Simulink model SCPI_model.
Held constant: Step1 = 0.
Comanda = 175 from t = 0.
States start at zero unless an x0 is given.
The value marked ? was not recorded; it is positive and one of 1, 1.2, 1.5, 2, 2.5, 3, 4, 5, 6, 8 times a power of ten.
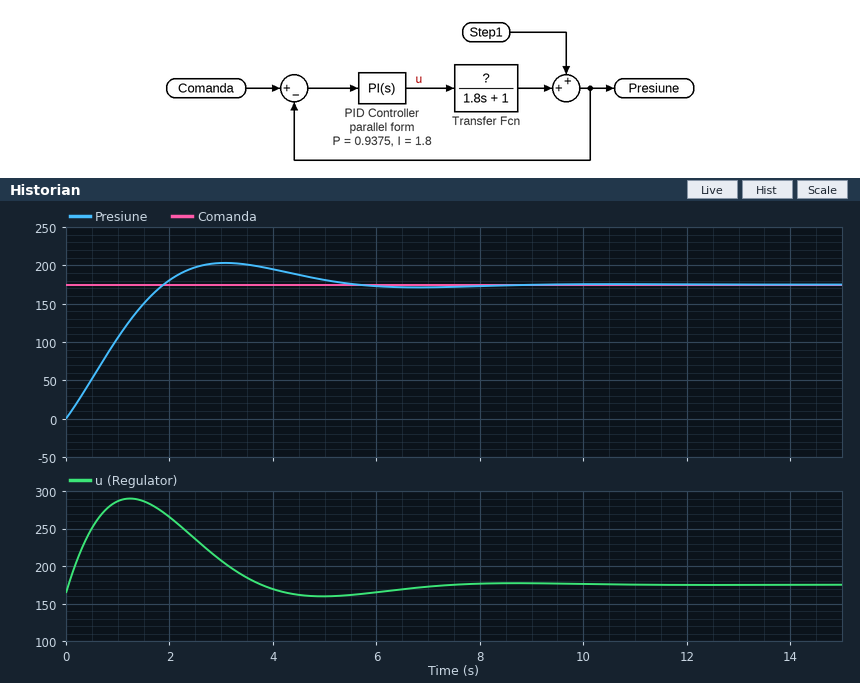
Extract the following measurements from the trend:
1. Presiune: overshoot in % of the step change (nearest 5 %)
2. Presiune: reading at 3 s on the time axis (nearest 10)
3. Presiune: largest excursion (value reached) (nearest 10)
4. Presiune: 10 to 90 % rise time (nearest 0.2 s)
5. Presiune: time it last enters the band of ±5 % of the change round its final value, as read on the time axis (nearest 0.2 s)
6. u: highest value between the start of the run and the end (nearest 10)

15 %
200
200
1.4 s
4.8 s
290
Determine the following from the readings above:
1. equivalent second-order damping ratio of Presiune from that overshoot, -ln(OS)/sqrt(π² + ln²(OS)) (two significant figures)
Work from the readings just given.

0.52
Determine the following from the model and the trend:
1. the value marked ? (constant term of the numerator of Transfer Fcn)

1
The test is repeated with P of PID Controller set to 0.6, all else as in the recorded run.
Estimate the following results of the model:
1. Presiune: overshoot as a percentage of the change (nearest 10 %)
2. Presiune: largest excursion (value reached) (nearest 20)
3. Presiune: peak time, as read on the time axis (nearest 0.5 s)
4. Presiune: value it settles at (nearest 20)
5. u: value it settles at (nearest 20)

20 %
220
3.0 s
180
180
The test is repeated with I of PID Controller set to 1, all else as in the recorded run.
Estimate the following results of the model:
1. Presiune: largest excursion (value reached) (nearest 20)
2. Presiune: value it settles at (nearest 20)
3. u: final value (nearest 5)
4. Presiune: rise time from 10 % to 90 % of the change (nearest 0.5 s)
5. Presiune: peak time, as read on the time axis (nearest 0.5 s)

180
180
175
2.0 s
4.5 s
